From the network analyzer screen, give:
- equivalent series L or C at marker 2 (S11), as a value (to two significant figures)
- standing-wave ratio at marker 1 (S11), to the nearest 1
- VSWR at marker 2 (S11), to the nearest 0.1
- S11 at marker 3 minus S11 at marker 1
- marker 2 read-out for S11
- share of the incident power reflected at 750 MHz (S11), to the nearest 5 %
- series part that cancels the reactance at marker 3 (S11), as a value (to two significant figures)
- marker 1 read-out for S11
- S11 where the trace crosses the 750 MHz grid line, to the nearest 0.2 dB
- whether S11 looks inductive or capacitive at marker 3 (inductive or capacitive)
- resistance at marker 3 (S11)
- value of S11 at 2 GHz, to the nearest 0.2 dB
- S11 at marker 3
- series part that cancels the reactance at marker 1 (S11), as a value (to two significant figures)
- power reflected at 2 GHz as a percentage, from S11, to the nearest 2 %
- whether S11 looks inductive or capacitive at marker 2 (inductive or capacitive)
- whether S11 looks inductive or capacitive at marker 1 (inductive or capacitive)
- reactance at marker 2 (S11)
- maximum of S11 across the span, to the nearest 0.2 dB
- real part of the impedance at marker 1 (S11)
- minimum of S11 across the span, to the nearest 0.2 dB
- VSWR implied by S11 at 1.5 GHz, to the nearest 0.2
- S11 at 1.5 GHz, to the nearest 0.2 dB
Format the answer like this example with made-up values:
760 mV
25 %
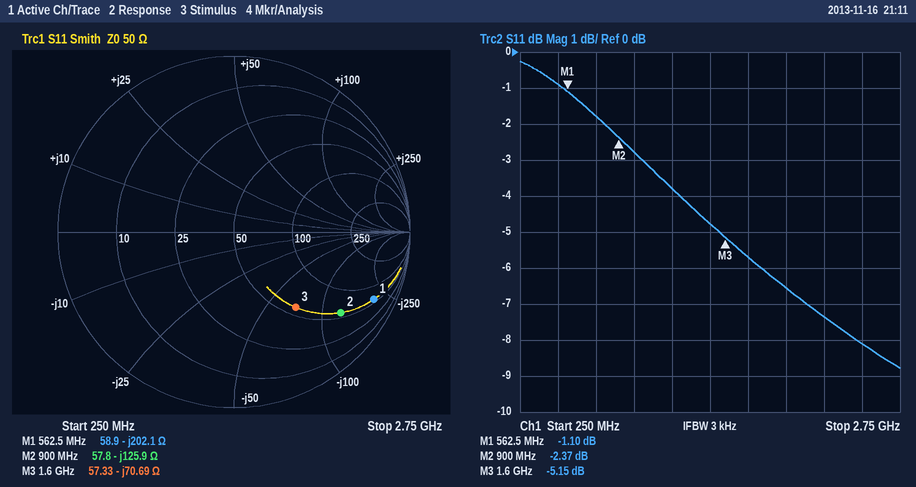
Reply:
1.4 pF
16
7.4
-4.05 dB
-2.37 dB
65 %
7.0 nH
-1.10 dB
-1.8 dB
capacitive
57.33 Ω
-6.6 dB
-5.15 dB
57 nH
22 %
capacitive
capacitive
-125.9 Ω
-0.2 dB
58.9 Ω
-8.8 dB
3.8
-4.8 dB
